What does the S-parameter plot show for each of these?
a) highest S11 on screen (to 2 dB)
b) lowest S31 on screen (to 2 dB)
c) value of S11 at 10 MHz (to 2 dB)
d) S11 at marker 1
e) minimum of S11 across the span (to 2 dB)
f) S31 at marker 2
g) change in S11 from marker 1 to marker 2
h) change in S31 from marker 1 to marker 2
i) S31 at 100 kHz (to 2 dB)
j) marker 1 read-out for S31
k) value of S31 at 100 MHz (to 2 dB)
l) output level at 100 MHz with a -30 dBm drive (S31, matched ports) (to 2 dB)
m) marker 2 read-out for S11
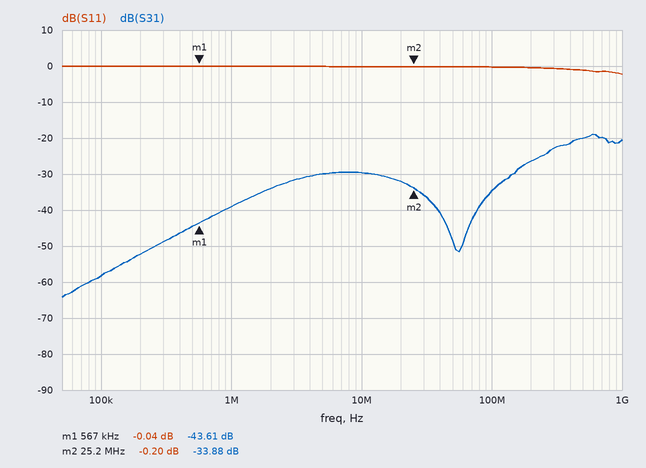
0 dB
-64 dB
0 dB
-0.04 dB
-2 dB
-33.88 dB
-0.16 dB
9.73 dB
-58 dB
-43.61 dB
-34 dB
-64 dBm
-0.20 dB
